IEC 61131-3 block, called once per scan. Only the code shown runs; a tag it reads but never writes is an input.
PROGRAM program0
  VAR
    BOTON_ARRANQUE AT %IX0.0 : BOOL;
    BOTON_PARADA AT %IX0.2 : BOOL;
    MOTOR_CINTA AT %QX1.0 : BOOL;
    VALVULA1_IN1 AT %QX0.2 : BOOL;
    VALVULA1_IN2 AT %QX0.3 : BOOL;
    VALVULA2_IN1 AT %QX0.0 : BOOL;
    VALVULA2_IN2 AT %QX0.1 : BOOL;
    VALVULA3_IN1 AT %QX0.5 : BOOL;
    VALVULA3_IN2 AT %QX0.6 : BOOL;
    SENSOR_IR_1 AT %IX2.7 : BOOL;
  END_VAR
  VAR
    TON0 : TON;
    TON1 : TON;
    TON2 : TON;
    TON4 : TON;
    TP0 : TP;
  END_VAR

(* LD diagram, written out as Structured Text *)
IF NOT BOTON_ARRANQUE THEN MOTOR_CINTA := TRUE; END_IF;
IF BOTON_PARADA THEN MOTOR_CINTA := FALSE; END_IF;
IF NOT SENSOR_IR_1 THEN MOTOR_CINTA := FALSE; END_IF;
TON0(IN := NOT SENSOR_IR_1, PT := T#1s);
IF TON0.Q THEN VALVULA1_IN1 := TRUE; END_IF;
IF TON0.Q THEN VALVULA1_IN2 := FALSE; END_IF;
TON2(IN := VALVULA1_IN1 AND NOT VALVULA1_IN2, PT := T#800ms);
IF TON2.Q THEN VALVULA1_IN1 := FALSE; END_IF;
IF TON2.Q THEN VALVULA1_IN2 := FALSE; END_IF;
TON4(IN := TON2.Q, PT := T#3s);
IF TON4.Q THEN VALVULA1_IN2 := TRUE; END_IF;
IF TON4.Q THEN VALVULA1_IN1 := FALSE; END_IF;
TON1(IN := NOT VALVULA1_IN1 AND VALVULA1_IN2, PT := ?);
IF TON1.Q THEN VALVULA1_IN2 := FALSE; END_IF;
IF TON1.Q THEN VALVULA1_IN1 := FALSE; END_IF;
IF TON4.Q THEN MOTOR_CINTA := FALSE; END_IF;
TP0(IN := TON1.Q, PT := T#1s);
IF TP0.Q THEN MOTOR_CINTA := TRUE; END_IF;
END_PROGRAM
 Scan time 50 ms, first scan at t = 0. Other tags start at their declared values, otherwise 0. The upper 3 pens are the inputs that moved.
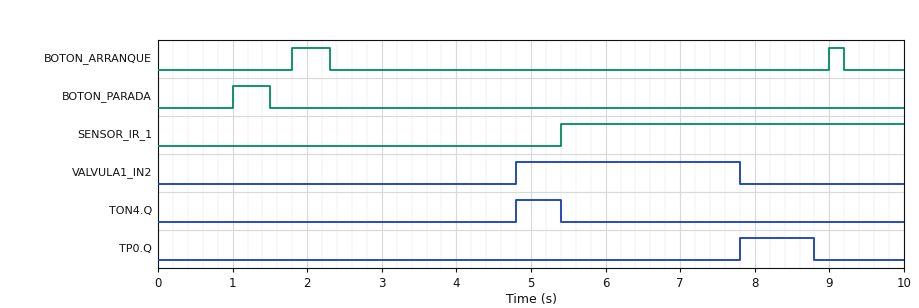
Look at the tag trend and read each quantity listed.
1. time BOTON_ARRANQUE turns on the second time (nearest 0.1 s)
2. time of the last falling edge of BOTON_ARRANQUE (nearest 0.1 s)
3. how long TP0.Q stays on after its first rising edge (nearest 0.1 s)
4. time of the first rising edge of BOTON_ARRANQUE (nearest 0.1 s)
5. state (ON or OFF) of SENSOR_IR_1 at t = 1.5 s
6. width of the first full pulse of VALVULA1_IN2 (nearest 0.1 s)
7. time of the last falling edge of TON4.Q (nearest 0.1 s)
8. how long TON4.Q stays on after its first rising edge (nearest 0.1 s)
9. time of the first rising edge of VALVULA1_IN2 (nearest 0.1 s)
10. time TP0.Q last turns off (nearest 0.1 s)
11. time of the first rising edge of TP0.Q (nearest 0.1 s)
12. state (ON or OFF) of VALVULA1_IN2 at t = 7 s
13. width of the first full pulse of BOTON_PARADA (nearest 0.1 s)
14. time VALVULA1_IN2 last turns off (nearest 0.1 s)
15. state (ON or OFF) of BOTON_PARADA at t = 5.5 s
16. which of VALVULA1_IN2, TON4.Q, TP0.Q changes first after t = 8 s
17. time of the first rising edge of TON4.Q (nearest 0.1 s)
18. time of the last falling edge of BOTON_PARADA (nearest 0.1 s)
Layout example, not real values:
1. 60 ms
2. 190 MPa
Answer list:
1. 9.0 s
2. 9.2 s
3. 1.0 s
4. 1.8 s
5. OFF
6. 3.0 s
7. 5.4 s
8. 0.6 s
9. 4.8 s
10. 8.8 s
11. 7.8 s
12. ON
13. 0.5 s
14. 7.8 s
15. OFF
16. TP0.Q
17. 4.8 s
18. 1.5 s
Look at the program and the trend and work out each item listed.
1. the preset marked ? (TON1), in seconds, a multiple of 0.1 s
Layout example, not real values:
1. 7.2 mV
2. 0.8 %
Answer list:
1. 3.0 s
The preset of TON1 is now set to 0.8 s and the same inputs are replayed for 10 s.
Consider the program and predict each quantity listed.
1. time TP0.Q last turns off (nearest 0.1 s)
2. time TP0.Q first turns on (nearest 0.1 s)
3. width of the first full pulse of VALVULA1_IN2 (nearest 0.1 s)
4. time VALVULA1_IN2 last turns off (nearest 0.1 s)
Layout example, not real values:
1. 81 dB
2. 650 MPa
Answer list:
1. 6.6 s
2. 5.6 s
3. 0.8 s
4. 5.6 s
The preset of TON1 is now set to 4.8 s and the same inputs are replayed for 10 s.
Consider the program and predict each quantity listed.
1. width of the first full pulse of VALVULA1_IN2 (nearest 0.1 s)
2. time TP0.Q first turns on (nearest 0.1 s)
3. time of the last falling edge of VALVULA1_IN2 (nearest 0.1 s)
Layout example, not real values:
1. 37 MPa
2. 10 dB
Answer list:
1. 4.8 s
2. 9.6 s
3. 9.6 s
